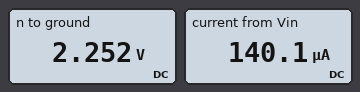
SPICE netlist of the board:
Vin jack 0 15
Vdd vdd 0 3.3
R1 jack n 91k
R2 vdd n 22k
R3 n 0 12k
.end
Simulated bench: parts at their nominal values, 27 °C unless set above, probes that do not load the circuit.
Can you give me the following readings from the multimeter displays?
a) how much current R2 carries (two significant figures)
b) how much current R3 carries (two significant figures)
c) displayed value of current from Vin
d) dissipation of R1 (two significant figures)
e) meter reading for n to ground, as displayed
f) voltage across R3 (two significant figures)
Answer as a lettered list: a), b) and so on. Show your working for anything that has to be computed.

a) (3.3 V - 2.252 V) / 22 kΩ = 48 µA
b) (2.252 V) / 12 kΩ = 190 µA
c) 140.1 µA
d) (15 V - 2.252 V)^2 / 91 kΩ = 1.8 mW
e) 2.252 V
f) 2.252 V = 2.3 V
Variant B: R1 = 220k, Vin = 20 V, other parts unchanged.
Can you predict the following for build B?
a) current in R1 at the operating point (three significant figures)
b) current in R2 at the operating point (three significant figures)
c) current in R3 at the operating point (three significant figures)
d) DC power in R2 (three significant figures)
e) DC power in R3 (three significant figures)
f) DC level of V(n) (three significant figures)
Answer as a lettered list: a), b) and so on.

a) 82.7 µA
b) 67.9 µA
c) 151 µA
d) 101 µW
e) 272 µW
f) 1.81 V
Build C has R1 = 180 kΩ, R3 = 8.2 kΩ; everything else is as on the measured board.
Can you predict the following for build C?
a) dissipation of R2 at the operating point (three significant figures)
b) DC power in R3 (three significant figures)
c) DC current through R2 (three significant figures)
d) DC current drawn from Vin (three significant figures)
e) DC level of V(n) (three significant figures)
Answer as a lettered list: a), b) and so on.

a) 173 µW
b) 222 µW
c) 88.7 µA
d) 75.8 µA
e) 1.35 V
